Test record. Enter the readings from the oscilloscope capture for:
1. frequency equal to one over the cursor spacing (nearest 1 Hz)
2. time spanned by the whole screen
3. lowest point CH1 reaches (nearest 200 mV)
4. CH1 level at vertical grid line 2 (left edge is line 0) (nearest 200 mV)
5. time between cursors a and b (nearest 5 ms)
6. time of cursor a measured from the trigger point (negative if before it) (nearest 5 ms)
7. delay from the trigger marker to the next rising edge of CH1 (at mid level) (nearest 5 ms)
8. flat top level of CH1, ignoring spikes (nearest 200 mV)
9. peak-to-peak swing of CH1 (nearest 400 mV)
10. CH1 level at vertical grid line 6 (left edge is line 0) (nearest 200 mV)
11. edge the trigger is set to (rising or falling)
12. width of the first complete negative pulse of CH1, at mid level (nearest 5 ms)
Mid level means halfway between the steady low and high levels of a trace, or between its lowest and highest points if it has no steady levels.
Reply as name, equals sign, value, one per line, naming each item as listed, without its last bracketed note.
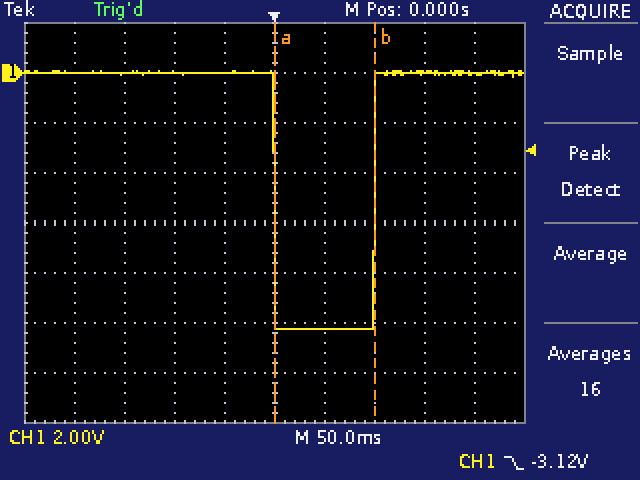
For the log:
frequency equal to one over the cursor spacing = 10 Hz
time spanned by the whole screen = 500 ms
lowest point CH1 reaches = -10.2 V
CH1 level at vertical grid line 2 (left edge is line 0) = 0.0 V
time between cursors a and b = 100 ms
time of cursor a measured from the trigger point (negative if before it) = 0 ms
delay from the trigger marker to the next rising edge of CH1 (at mid level) = 100 ms
flat top level of CH1, ignoring spikes = 0.0 V
peak-to-peak swing of CH1 = 10.4 V
CH1 level at vertical grid line 6 (left edge is line 0) = -10.2 V
edge the trigger is set to = falling
width of the first complete negative pulse of CH1, at mid level = 100 ms
